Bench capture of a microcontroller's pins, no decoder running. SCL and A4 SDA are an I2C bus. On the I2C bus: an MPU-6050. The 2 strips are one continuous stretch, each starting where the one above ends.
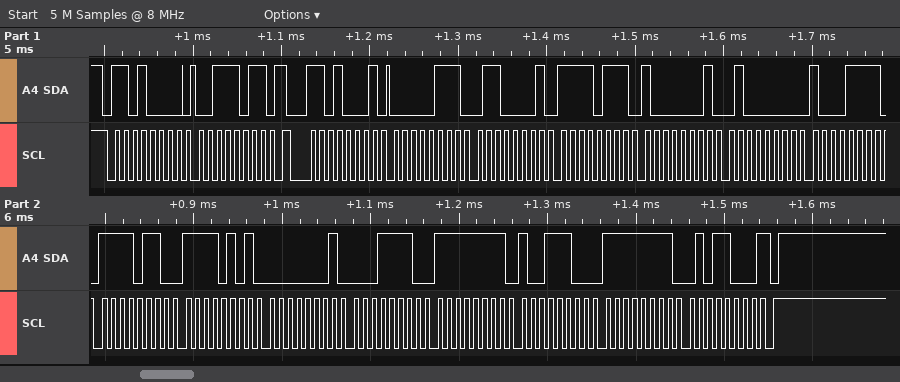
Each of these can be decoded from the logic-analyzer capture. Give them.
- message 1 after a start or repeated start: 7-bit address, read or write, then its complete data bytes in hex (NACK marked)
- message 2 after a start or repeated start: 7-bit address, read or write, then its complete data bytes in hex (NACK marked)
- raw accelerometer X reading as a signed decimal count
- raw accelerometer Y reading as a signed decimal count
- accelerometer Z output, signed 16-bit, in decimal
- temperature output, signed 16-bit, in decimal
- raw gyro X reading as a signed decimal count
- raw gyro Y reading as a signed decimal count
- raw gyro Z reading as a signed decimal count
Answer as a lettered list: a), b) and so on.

a) 0x68 write: 3B
b) 0x68 read: 07 61 F7 81 40 8F F6 F5 01 1E FF 9C FF 58 NACK
c) 1889
d) -2175
e) 16527
f) -2315
g) 286
h) -100
i) -168
